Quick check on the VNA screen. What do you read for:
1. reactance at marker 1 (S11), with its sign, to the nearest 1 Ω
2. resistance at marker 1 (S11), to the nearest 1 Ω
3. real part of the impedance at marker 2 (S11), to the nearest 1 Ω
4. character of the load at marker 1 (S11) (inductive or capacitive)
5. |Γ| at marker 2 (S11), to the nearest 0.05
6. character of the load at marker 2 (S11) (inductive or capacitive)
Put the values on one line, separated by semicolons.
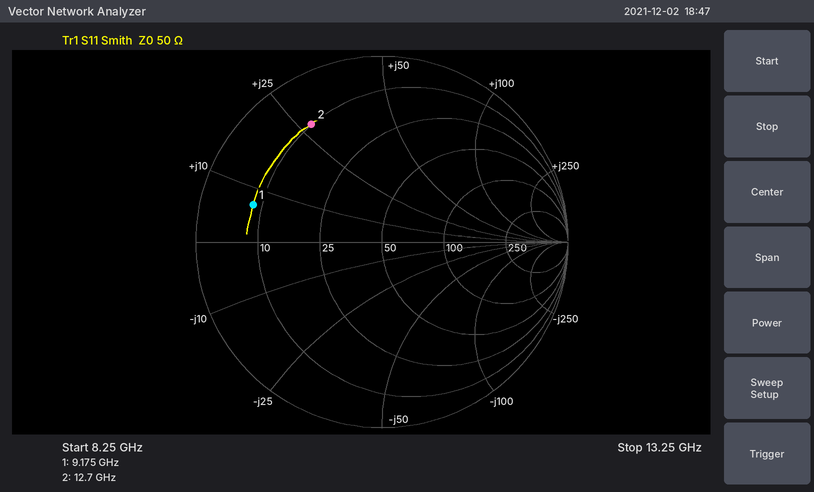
+7 Ω; 8 Ω; 10 Ω; inductive; 0.75; inductive
